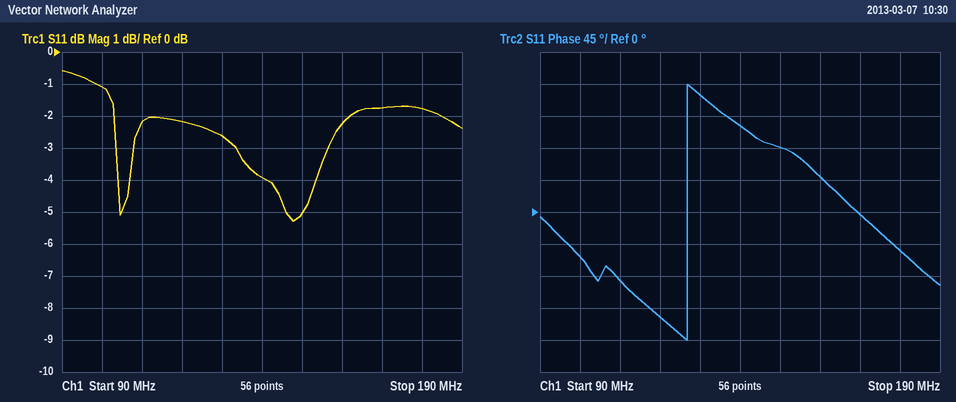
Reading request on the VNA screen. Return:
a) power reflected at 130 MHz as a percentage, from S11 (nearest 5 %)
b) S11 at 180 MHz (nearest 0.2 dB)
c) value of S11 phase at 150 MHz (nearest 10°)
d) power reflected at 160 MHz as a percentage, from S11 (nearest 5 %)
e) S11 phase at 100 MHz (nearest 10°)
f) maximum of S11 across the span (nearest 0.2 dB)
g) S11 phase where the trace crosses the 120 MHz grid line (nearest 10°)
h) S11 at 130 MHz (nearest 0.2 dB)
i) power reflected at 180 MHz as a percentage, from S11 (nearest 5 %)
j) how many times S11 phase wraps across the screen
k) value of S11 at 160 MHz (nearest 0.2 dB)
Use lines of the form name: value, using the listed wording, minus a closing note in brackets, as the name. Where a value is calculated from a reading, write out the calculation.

power reflected at 130 MHz as a percentage, from S11: 10^(-2.6/10) ≈ 55 %
S11 at 180 MHz: -1.8 dB
value of S11 phase at 150 MHz: 90°
power reflected at 160 MHz as a percentage, from S11: 10^(-2.2/10) ≈ 60 %
S11 phase at 100 MHz: -60°
maximum of S11 across the span: -0.6 dB
S11 phase where the trace crosses the 120 MHz grid line: -150°
S11 at 130 MHz: -2.6 dB
power reflected at 180 MHz as a percentage, from S11: 10^(-1.8/10) ≈ 66.1 %, so 65 % to the nearest 5 %
how many times S11 phase wraps across the screen: 1
value of S11 at 160 MHz: -2.2 dB
